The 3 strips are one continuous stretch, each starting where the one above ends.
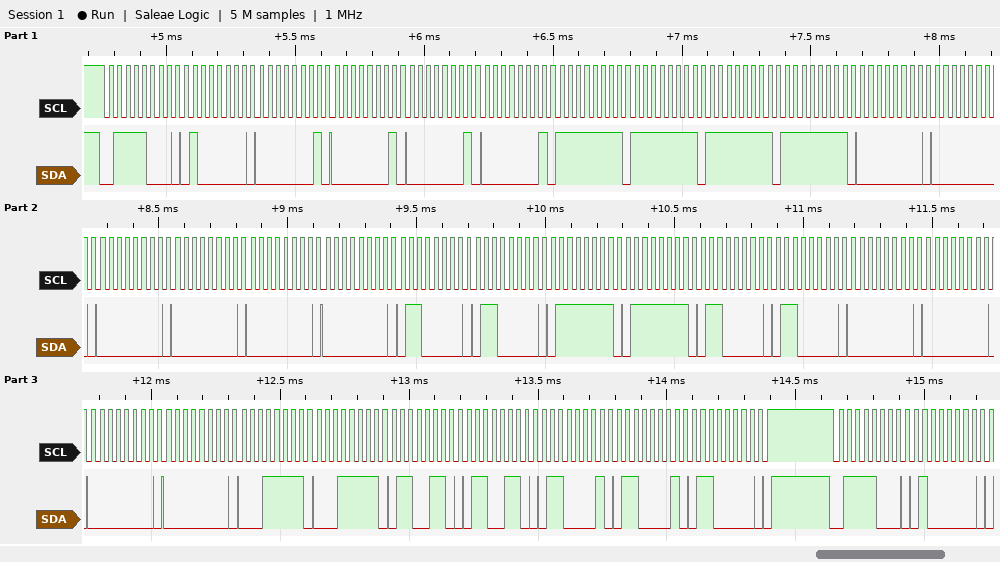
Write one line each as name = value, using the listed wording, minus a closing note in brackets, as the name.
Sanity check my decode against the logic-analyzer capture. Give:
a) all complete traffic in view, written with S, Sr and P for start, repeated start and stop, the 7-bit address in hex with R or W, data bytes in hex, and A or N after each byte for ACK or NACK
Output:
all complete traffic in view, written with S, Sr and P for start, repeated start and stop, the 7-bit address in hex with R or W, data bytes in hex, and A or N after each byte for ACK or NACK = S 3CW A 40 A 01 A 01 A 01 A 01 A FF A FF A FF A FF A 00 A 00 A 00 A 00 A 00 A 00 A 60 A 60 A 7F A 7F A 60 A 60 A 00 A 00 A 00 A 00 A 1F A 1F A 66 A 66 A 61 A 61 A 60 A P S 3CW A 40 A
